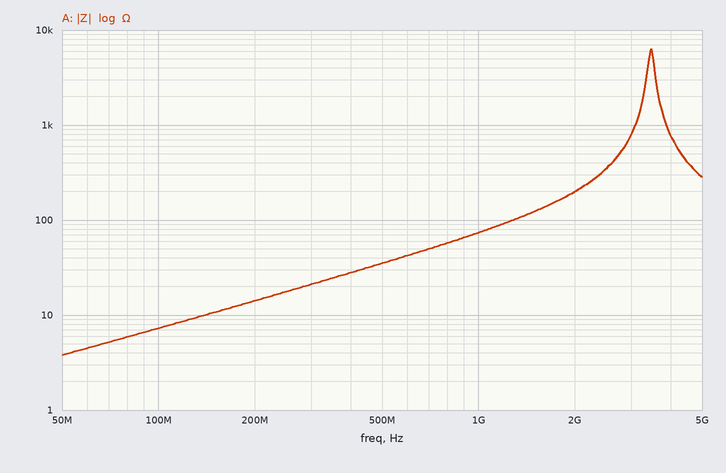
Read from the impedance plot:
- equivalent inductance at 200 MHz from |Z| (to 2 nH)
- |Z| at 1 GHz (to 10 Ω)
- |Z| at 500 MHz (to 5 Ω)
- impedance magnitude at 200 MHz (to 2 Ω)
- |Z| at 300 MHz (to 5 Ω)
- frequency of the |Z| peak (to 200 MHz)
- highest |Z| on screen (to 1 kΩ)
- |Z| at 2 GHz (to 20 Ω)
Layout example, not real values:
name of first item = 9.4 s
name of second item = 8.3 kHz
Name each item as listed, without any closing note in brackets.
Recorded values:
equivalent inductance at 200 MHz from |Z| = 12 nH
|Z| at 1 GHz = 70 Ω
|Z| at 500 MHz = 35 Ω
impedance magnitude at 200 MHz = 14 Ω
|Z| at 300 MHz = 20 Ω
frequency of the |Z| peak = 3.4 GHz
highest |Z| on screen = 6 kΩ
|Z| at 2 GHz = 200 Ω
